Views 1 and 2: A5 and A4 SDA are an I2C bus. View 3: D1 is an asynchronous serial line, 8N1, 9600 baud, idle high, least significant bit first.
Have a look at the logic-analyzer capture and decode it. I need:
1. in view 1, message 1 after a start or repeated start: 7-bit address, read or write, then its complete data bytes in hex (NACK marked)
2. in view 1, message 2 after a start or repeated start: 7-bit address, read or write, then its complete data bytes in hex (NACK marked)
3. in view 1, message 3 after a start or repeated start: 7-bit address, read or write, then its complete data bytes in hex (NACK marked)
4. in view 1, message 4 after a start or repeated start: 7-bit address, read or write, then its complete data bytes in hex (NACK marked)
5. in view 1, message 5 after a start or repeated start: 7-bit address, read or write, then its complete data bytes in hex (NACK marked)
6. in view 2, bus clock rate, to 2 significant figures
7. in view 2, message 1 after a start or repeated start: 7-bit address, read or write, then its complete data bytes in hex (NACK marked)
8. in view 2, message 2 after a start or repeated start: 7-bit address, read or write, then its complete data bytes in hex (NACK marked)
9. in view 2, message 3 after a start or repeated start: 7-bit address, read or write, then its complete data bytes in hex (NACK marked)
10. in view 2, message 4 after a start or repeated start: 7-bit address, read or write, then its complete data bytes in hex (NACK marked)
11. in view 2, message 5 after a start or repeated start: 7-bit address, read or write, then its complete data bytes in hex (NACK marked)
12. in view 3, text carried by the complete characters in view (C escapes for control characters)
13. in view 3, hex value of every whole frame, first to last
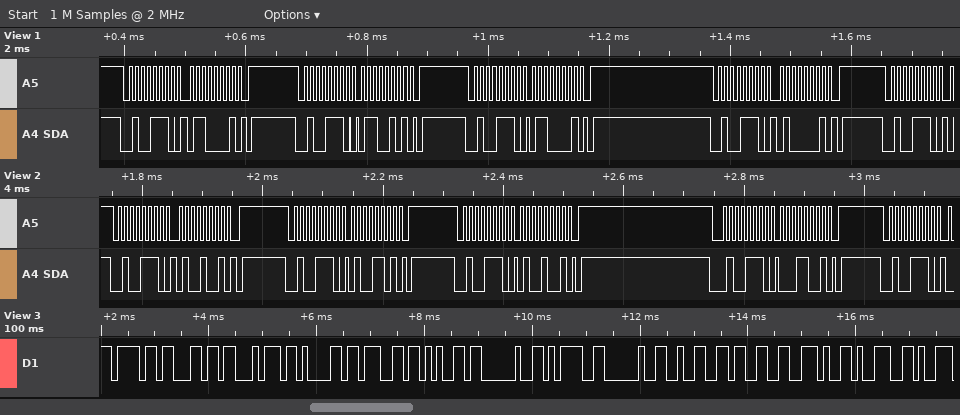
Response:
0x27 write: 61
0x27 write: 65
0x27 write: 61
0x27 write: 41
0x27 write
100 kHz
0x27 write: 49
0x27 write: 4D
0x27 write: 49
0x27 write: 19
0x27 write
"oltage = 23.9"
6F 6C 74 61 67 65 20 3D 20 32 33 2E 39
